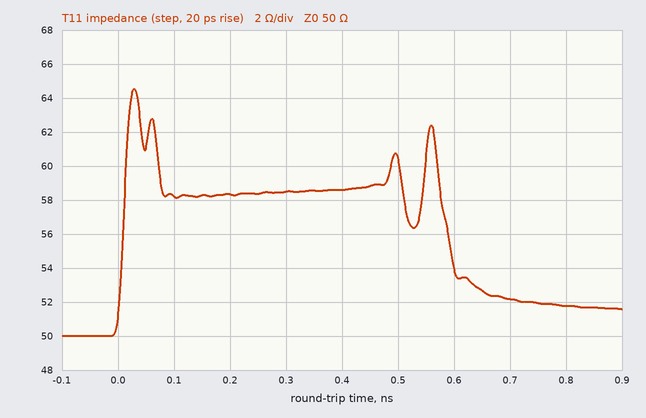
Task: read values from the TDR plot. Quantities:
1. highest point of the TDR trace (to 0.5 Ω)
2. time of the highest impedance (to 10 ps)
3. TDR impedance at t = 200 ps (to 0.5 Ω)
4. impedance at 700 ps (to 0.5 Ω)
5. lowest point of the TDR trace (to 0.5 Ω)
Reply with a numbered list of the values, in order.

1. 64.5 Ω
2. 30 ps
3. 58.5 Ω
4. 52.0 Ω
5. 50.0 Ω
